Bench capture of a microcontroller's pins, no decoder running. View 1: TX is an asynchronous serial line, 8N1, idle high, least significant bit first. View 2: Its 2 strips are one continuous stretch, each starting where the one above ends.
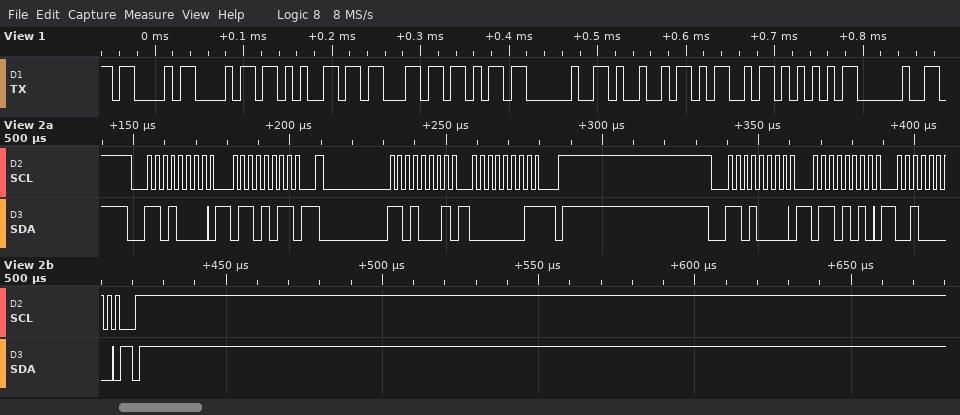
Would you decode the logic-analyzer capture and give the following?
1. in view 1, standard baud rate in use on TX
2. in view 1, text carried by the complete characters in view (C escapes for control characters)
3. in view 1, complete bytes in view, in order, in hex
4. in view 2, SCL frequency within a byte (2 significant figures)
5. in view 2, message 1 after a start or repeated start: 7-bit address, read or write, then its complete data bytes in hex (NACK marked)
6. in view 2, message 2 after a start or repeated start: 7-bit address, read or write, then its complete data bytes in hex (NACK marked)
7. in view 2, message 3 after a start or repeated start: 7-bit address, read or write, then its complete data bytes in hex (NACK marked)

115200 baud
"Check IMU "
43 68 65 63 6B 20 49 4D 55 20
400 kHz
0x68 write: 6B
0x68 read: 01 NACK
0x68 write: 6A 20
